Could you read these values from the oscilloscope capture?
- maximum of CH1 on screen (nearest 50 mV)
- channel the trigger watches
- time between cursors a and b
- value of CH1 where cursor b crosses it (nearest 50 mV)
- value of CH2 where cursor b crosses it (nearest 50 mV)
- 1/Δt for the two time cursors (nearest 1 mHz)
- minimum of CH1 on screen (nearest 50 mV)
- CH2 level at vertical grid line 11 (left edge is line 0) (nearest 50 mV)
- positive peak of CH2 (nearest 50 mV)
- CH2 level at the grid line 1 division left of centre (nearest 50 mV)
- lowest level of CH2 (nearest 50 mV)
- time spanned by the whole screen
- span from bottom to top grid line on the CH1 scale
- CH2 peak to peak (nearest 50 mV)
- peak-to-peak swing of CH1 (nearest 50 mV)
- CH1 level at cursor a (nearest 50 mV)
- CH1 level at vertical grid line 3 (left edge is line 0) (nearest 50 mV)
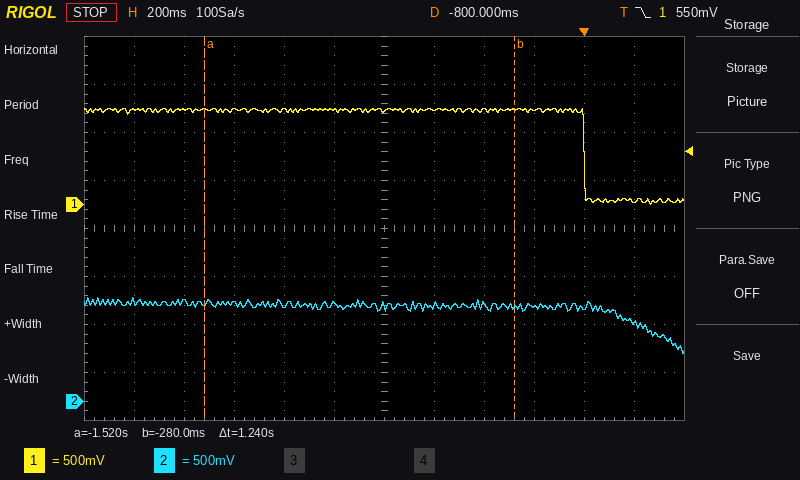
1.00 V
CH1
1.24 s
1.00 V
1.00 V
806 mHz
0 mV
800 mV
1.10 V
1.00 V
500 mV
2.4 s
4 V
600 mV
1.00 V
1.00 V
1.00 V
